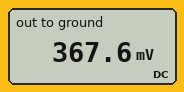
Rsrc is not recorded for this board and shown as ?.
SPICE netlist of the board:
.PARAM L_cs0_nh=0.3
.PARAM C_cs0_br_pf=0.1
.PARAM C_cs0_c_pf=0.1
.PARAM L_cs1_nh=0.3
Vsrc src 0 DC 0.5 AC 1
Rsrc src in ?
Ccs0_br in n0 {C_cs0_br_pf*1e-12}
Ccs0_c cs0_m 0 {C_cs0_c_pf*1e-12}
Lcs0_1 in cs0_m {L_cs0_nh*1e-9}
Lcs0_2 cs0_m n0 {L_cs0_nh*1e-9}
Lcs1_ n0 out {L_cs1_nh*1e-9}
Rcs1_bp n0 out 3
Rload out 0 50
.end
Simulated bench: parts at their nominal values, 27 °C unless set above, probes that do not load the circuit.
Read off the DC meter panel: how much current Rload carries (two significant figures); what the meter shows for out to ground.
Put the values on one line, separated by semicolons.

7.4 mA; 367.6 mV
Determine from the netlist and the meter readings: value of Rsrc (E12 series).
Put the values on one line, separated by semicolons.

18 Ω
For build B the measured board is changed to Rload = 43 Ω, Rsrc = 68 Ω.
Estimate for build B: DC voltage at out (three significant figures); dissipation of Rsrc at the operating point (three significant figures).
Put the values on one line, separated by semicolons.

194 mV; 1.38 mW
